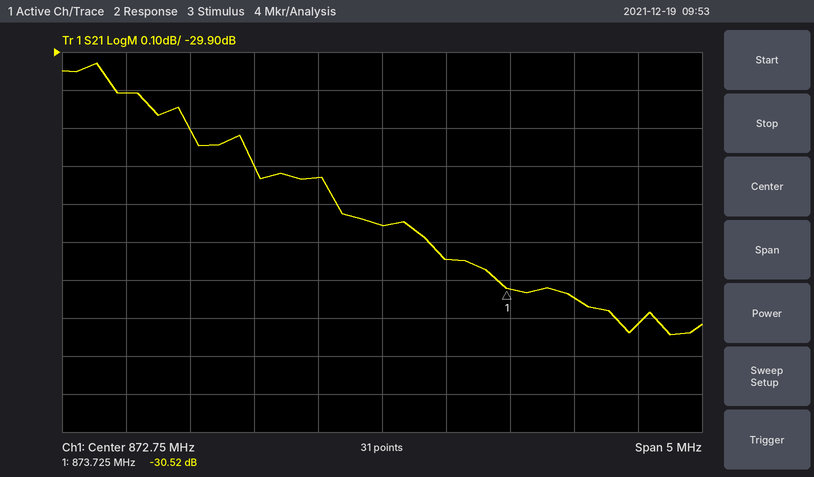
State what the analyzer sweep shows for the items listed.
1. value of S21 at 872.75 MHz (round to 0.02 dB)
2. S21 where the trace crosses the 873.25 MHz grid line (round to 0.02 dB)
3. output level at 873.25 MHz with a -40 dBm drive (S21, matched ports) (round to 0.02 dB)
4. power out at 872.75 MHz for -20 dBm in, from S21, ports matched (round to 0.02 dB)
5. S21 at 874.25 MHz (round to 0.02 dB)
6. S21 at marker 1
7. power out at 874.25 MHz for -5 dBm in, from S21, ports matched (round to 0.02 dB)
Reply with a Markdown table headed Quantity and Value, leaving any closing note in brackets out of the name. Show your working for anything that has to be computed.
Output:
| Quantity | Value |
|---|---|
| value of S21 at 872.75 MHz | -30.36 dB |
| S21 where the trace crosses the 873.25 MHz grid line | -30.44 dB |
| output level at 873.25 MHz with a -40 dBm drive (S21, matched ports) | -40 dBm + (-30.44 dB) = -70.44 dBm |
| power out at 872.75 MHz for -20 dBm in, from S21, ports matched | -20 dBm + (-30.36 dB) = -50.36 dBm |
| S21 at 874.25 MHz | -30.54 dB |
| S21 at marker 1 | -30.52 dB |
| power out at 874.25 MHz for -5 dBm in, from S21, ports matched | -5 dBm + (-30.54 dB) = -35.54 dBm |
